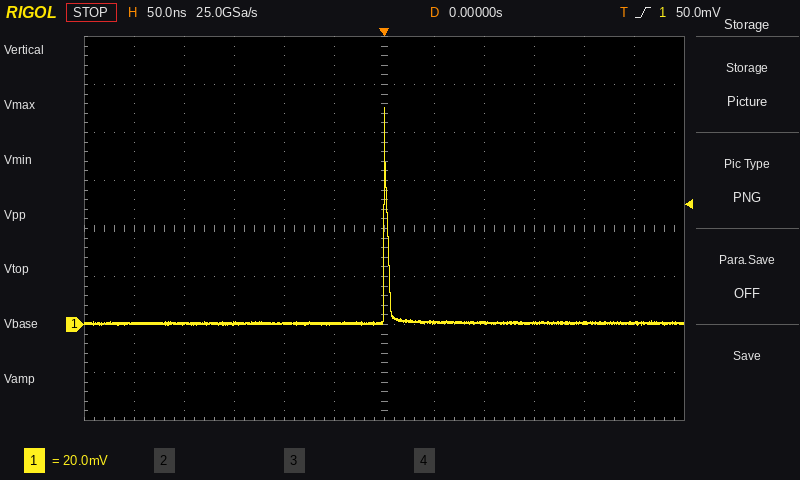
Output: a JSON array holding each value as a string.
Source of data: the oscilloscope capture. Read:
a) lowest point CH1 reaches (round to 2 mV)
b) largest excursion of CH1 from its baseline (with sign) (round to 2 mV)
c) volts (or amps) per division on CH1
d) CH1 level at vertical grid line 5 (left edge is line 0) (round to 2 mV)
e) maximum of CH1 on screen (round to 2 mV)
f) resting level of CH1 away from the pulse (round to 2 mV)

["0 mV", "+90 mV", "20 mV", "0 mV", "90 mV", "0 mV"]
